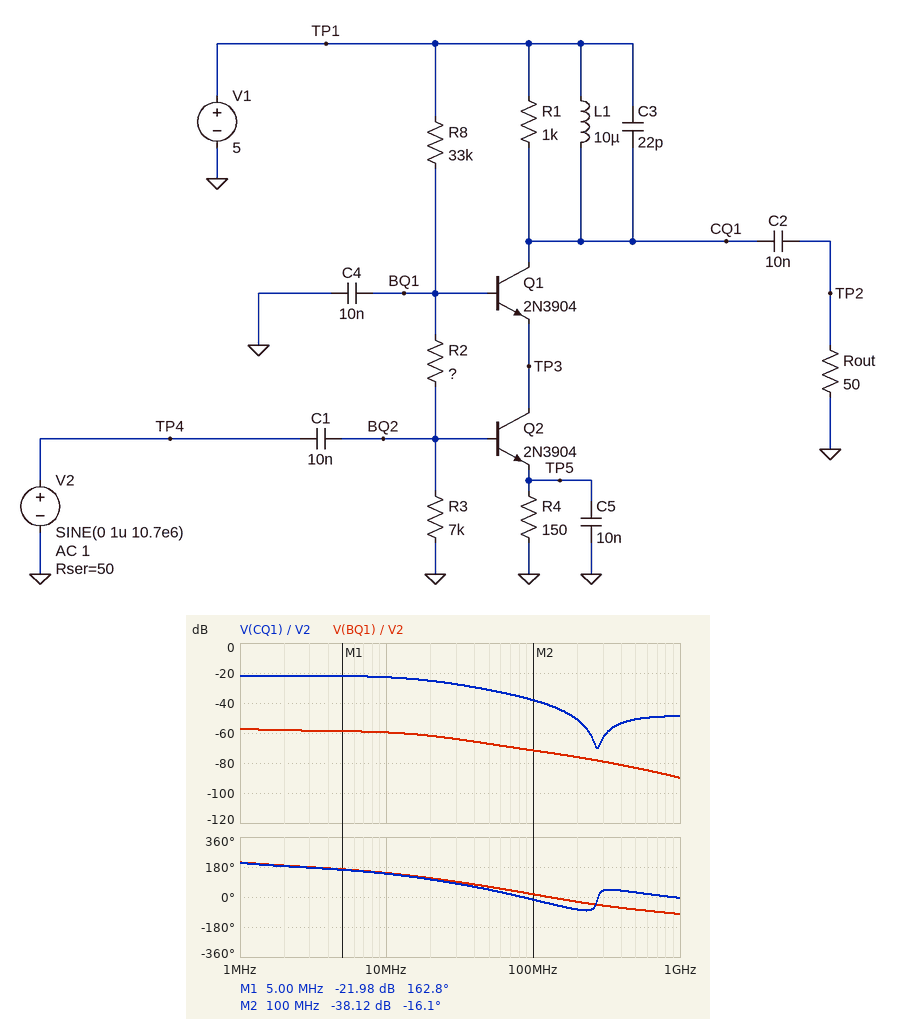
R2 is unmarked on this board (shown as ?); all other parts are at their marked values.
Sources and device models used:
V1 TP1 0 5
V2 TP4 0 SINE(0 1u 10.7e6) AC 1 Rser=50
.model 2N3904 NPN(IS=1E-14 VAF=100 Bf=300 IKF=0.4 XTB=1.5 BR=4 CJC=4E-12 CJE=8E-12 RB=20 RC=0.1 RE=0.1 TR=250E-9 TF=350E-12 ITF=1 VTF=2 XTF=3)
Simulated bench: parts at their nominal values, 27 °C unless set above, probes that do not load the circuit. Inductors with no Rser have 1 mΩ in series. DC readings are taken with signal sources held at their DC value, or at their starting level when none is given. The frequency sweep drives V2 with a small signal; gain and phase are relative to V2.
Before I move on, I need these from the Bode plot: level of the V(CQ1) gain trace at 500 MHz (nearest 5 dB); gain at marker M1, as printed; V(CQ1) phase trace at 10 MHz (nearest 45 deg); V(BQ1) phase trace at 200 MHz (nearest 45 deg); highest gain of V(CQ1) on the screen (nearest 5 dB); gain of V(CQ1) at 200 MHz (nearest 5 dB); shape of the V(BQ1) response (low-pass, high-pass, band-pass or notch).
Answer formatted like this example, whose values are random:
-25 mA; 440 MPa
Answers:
-50 dB; -21.98 dB; 135 deg; -45 deg; -20 dB; -50 dB; low-pass
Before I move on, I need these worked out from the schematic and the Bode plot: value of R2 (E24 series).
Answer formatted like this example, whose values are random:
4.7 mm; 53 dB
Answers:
20 kΩ
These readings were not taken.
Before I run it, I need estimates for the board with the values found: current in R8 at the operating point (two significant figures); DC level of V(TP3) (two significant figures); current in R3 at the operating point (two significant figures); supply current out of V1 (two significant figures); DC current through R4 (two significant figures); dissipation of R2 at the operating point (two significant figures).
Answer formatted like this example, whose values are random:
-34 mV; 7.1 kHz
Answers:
83 µA; 1.7 V; 83 µA; 130 µA; 46 µA; 140 µW
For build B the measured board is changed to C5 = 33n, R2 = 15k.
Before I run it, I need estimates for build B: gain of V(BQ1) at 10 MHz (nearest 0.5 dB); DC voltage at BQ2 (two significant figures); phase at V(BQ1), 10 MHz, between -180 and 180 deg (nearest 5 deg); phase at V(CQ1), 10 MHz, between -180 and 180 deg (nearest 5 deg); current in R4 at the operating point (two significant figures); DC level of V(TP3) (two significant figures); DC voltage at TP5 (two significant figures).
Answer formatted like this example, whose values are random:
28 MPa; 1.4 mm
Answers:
-57.0 dB; 630 mV; 165 deg; 160 deg; 160 µA; 1.4 V; 24 mV
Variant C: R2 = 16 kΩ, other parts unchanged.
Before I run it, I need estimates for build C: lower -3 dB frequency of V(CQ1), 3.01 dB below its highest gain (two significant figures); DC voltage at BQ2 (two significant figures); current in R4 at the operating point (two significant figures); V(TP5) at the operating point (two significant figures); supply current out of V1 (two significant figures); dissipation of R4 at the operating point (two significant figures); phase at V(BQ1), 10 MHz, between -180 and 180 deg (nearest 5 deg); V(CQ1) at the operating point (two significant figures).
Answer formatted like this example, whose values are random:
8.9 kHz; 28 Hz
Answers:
470 kHz; 620 mV; 130 µA; 19 mV; 220 µA; 2.4 µW; 165 deg; 5.0 V
